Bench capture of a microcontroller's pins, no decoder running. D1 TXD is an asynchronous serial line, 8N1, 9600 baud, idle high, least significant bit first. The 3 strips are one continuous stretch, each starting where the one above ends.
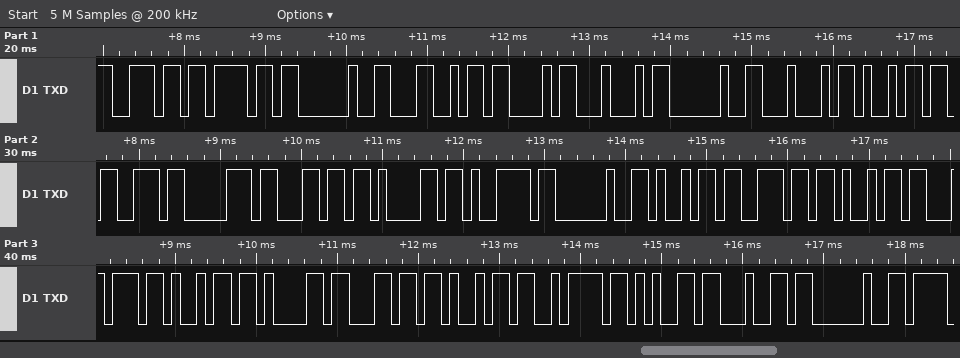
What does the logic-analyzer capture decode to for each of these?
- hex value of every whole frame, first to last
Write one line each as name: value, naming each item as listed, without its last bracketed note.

hex value of every whole frame, first to last: 6E 6F 20 4C 43 44 20 44 69 73 70 6C 61 79 20 69 6E 69 74 69 61 6C 69 7A 65 64 20
